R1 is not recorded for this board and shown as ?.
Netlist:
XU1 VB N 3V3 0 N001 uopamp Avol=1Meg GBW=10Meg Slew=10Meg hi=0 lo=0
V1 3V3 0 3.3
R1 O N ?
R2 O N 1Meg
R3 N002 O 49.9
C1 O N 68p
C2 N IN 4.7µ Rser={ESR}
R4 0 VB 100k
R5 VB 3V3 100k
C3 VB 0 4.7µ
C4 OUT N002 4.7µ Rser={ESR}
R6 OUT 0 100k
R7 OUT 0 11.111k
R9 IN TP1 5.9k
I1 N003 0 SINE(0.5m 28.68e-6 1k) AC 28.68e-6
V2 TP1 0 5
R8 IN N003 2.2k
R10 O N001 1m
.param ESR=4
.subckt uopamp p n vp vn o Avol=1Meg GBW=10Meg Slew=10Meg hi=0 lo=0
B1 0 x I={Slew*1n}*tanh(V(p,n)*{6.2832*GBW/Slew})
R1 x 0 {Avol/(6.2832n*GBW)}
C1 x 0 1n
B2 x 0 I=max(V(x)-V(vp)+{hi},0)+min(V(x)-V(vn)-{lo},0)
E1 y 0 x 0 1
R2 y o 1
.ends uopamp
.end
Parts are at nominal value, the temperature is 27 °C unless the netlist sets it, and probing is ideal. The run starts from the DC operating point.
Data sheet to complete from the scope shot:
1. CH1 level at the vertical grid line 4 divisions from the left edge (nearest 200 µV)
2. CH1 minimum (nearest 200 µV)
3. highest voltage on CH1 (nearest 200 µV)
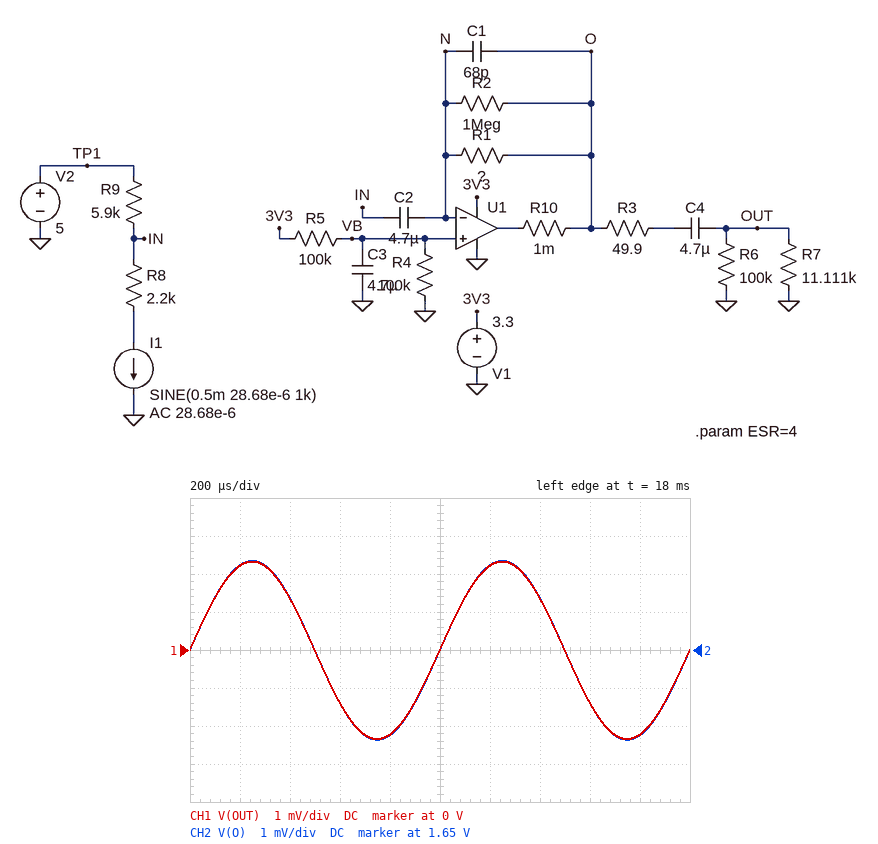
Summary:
-2.2 mV
-2.4 mV
2.4 mV
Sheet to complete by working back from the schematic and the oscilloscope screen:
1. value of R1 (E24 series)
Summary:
82 Ω
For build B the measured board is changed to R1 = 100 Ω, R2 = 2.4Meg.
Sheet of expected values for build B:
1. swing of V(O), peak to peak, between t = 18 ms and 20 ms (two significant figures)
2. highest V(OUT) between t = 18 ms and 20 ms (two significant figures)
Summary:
5.7 mV
2.8 mV
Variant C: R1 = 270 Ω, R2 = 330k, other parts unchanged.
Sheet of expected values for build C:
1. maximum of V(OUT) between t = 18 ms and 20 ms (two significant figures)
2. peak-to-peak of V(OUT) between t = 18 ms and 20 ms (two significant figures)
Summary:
7.7 mV
15 mV
